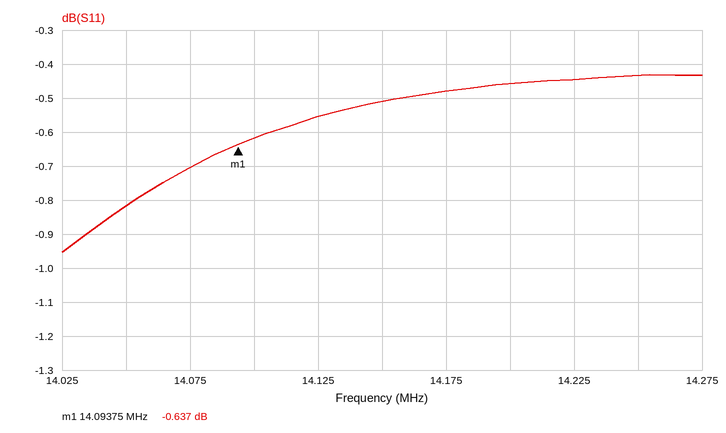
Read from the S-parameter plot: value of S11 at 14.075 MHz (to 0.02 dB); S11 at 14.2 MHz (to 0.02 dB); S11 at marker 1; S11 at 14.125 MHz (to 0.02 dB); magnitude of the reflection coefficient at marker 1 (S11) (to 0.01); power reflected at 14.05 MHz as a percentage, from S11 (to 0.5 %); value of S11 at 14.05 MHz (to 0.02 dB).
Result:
-0.70 dB
-0.46 dB
-0.637 dB
-0.56 dB
0.93
83.0 %
-0.82 dB
